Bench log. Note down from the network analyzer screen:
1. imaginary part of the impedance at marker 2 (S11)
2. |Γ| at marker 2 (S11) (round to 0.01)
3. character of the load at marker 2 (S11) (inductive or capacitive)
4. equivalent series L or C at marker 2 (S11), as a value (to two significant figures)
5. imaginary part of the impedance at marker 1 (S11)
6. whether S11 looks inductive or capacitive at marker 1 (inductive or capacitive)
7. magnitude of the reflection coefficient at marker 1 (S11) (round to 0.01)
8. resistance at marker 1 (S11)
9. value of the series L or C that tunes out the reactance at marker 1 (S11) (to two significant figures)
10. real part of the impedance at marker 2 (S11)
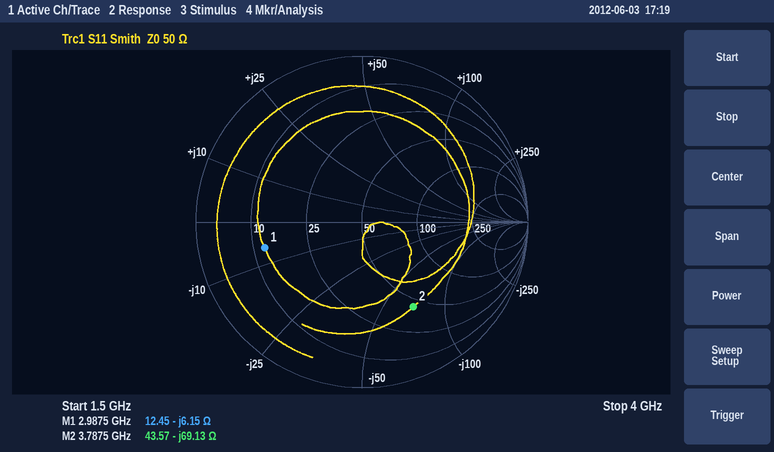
-69.13 Ω
0.60
capacitive
610 fF
-6.15 Ω
capacitive
0.61
12.45 Ω
330 pH
43.57 Ω
